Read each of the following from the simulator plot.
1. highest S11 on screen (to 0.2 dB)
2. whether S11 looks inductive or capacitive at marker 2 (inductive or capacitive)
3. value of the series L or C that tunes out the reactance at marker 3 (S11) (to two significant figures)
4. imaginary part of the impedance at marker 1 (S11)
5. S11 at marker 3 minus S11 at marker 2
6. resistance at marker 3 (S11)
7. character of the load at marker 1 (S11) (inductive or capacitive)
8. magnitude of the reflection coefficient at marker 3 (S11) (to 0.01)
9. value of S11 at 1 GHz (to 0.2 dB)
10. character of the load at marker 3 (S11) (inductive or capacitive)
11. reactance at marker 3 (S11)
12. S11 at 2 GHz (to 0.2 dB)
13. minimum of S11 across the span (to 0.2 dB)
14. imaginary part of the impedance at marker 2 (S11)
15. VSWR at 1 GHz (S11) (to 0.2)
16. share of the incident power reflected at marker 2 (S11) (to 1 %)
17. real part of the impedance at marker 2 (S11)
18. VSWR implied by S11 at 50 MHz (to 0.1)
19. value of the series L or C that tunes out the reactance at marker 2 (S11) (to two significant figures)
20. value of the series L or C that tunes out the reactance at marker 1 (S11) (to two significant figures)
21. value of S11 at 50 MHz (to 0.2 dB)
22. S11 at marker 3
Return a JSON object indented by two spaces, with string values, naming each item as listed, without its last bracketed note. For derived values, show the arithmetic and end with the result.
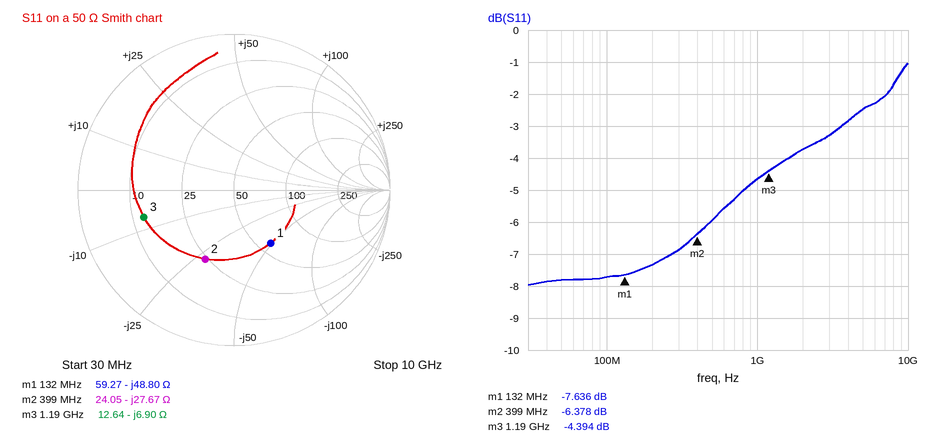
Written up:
{
  "highest S11 on screen": "-1.0 dB",
  "whether S11 looks inductive or capacitive at marker 2": "capacitive",
  "value of the series L or C that tunes out the reactance at marker 3 (S11)": "L = 6.9 Ω/(2π × 1.19 GHz) ≈ 923 pH, so 920 pH to two significant figures",
  "imaginary part of the impedance at marker 1": "-48.80 Ω",
  "S11 at marker 3 minus S11 at marker 2": "-4.394 − (-6.378) = 1.984 dB",
  "resistance at marker 3": "12.64 Ω",
  "character of the load at marker 1 (S11)": "capacitive",
  "magnitude of the reflection coefficient at marker 3 (S11)": "0.60",
  "value of S11 at 1 GHz": "-4.6 dB",
  "character of the load at marker 3 (S11)": "capacitive",
  "reactance at marker 3": "-6.90 Ω",
  "S11 at 2 GHz": "-3.8 dB",
  "minimum of S11 across the span": "-8.0 dB",
  "imaginary part of the impedance at marker 2": "-27.67 Ω",
  "VSWR at 1 GHz (S11)": "|Γ| = 10^(-4.6/20) = 0.5888; VSWR = (1 + 0.5888)/(1 − 0.5888) ≈ 3.86, so 3.8 to the nearest 0.2",
  "share of the incident power reflected at marker 2 (S11)": "10^(-6.378/10) ≈ 23 %",
  "real part of the impedance at marker 2": "24.05 Ω",
  "VSWR implied by S11 at 50 MHz": "|Γ| = 10^(-7.8/20) = 0.4074; VSWR = (1 + 0.4074)/(1 − 0.4074) ≈ 2.4",
  "value of the series L or C that tunes out the reactance at marker 2 (S11)": "L = 27.67 Ω/(2π × 399 MHz) ≈ 11 nH",
  "value of the series L or C that tunes out the reactance at marker 1 (S11)": "L = 48.8 Ω/(2π × 132 MHz) ≈ 59 nH",
  "value of S11 at 50 MHz": "-7.8 dB",
  "S11 at marker 3": "-4.394 dB"
}
